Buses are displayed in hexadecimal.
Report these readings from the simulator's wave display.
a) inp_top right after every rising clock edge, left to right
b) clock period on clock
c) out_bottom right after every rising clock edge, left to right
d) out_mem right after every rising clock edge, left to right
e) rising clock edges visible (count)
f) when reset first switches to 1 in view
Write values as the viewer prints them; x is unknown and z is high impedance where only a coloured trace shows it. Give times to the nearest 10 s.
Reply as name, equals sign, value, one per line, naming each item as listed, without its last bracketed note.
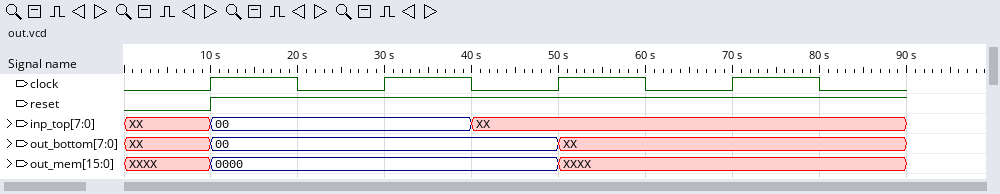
inp_top right after every rising clock edge, left to right = 00, 00, XX, XX
clock period on clock = 20 s
out_bottom right after every rising clock edge, left to right = 00, 00, XX, XX
out_mem right after every rising clock edge, left to right = 0000, 0000, XXXX, XXXX
rising clock edges visible = 4
when reset first switches to 1 in view = 10 s
